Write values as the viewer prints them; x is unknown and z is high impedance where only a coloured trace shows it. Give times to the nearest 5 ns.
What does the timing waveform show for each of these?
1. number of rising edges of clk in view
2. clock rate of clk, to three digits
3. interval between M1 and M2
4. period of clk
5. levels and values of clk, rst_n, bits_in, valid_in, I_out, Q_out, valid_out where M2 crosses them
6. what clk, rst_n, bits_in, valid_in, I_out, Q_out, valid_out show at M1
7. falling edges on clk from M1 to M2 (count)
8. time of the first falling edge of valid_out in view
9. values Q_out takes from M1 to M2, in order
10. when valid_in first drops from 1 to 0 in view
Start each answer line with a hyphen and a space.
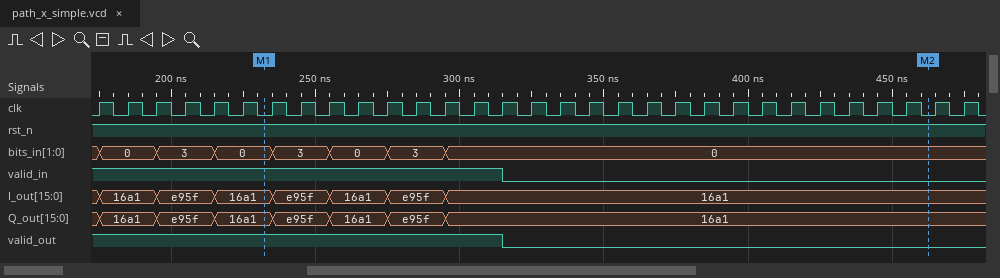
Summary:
- 31
- 100 MHz
- 230 ns
- 10 ns
- clk=0, rst_n=1, bits_in=0, valid_in=0, I_out=16a1, Q_out=16a1, valid_out=0
- clk=0, rst_n=1, bits_in=0, valid_in=1, I_out=16a1, Q_out=16a1, valid_out=1
- 23
- 315 ns
- 16a1, e95f, 16a1, e95f, 16a1
- 315 ns
